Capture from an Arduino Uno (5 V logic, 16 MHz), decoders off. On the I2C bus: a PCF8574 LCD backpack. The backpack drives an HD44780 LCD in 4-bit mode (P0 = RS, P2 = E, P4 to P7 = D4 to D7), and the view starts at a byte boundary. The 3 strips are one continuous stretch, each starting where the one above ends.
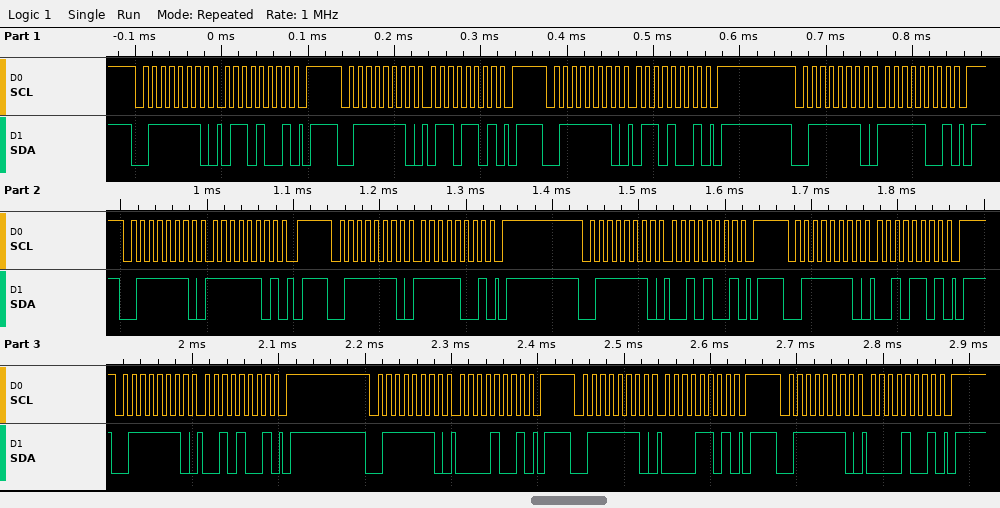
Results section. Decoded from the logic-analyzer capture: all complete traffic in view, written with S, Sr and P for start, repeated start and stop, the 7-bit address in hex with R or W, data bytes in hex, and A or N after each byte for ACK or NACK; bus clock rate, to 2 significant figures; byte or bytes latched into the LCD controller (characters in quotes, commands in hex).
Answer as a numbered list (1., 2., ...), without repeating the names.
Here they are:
1. S 3FW A 69 A P S 3FW A 6D A P S 3FW A 69 A P S 3FW A F9 A P S 3FW A FD A P S 3FW A F9 A P S 3FW A 29 A P S 3FW A 2D A P S 3FW A 29 A P S 3FW A 09 A P S 3FW A 0D A P S 3FW A 09 A P
2. 100 kHz
3. 'o' ' '
